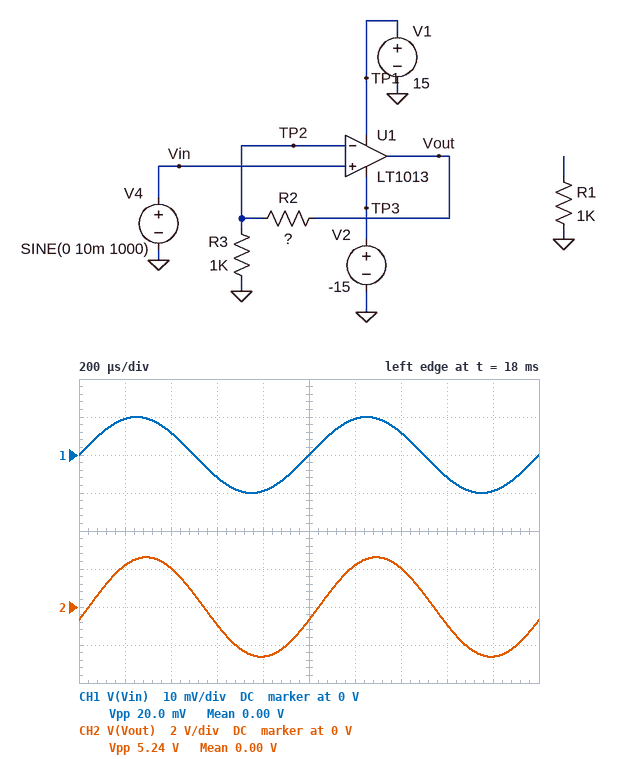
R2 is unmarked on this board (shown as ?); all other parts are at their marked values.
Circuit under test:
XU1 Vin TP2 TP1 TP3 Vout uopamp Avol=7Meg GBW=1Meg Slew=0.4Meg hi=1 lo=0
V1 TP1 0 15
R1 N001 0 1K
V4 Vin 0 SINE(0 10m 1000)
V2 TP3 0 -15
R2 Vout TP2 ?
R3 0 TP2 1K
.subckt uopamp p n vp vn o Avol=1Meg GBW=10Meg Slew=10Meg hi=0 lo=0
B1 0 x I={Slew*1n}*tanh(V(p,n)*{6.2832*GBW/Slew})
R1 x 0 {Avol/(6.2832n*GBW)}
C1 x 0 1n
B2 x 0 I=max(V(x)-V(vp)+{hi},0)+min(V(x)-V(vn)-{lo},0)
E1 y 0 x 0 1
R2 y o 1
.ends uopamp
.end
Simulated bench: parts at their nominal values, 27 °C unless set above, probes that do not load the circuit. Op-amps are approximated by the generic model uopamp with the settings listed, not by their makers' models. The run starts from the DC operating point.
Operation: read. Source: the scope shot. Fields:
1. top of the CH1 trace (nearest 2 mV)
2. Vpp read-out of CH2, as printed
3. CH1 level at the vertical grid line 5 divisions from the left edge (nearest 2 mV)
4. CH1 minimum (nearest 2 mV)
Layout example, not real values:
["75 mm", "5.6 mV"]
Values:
["10 mV", "5.24 V", "0 V", "-10 mV"]
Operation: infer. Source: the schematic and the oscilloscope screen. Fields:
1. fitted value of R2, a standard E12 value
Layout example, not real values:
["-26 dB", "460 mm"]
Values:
["270 kΩ"]
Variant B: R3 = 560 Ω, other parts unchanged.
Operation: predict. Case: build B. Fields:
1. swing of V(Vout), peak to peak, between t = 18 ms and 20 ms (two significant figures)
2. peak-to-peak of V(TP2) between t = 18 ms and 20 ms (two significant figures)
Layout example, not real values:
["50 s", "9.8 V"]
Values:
["8.7 V", "18 mV"]
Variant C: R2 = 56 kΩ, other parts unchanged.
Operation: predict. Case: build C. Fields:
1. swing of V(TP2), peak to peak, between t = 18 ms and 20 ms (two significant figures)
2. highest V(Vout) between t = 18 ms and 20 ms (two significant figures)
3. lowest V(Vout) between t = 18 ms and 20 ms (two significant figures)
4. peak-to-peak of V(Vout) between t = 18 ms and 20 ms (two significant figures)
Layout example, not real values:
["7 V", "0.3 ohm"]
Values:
["20 mV", "570 mV", "-570 mV", "1.1 V"]
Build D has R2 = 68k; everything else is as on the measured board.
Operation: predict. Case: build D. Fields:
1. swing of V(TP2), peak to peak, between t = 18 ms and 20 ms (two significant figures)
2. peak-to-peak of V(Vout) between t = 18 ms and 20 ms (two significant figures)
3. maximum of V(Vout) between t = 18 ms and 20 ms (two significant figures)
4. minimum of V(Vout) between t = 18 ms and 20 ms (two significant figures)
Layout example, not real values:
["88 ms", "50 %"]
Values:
["20 mV", "1.4 V", "690 mV", "-690 mV"]
